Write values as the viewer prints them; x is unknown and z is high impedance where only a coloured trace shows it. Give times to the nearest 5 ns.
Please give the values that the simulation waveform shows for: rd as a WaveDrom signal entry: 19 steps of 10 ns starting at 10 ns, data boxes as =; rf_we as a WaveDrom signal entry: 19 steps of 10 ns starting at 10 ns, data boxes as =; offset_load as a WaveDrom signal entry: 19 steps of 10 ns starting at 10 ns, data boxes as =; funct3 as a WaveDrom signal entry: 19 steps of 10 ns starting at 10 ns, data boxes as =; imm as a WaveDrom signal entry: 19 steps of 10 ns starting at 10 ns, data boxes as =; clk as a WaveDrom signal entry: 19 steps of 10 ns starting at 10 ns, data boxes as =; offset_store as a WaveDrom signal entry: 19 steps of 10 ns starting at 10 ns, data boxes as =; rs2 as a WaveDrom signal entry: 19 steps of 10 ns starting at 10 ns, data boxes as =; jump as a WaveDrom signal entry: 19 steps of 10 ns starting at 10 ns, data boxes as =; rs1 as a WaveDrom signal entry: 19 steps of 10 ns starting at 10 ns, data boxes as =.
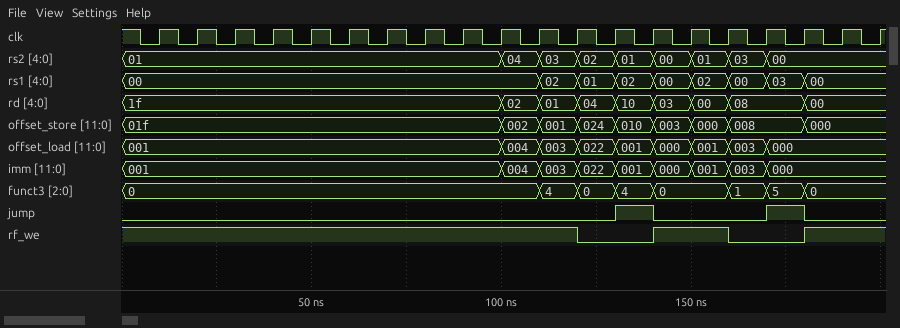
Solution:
{name: 'rd', wave: '=........=======.=.', data: '1f 02 01 04 10 03 00 08 00'}
{name: 'rf_we', wave: '1..........0.1.0.1.'}
{name: 'offset_load', wave: '=........========..', data: '001 004 003 022 001 000 001 003 000'}
{name: 'funct3', wave: '=.........====.===.', data: '0 4 0 4 0 1 5 0'}
{name: 'imm', wave: '=........========..', data: '001 004 003 022 001 000 001 003 000'}
{name: 'clk', wave: 'p..................'}
{name: 'offset_store', wave: '=........=======.=.', data: '01f 002 001 024 010 003 000 008 000'}
{name: 'rs2', wave: '=........========..', data: '01 04 03 02 01 00 01 03 00'}
{name: 'jump', wave: '0...........10..10.'}
{name: 'rs1', wave: '=.........========.', data: '00 02 01 02 00 02 00 03 00'}
